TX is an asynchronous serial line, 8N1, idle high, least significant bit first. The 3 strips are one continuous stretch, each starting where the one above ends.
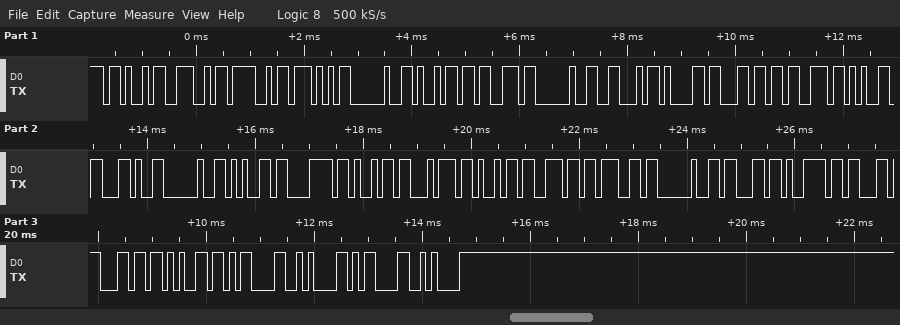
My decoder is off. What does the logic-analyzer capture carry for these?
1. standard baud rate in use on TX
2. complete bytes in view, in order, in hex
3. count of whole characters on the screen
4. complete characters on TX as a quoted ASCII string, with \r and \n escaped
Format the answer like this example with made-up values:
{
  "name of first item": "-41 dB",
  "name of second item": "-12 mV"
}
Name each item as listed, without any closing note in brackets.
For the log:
{
  "standard baud rate in use on TX": "9600 baud",
  "complete bytes in view, in order, in hex": "4B 4E 4F 57 20 69 73 20 46 61 6C 73 65 2C 20 65 78 69 74 69 6E 67 20 63 79 63 6C 65 0D 0A 0D 0A",
  "count of whole characters on the screen": "32",
  "complete characters on TX as a quoted ASCII string, with \\r and \\n escaped": "\"KNOW is False, exiting cycle\\r\\n\\r\\n\""
}
